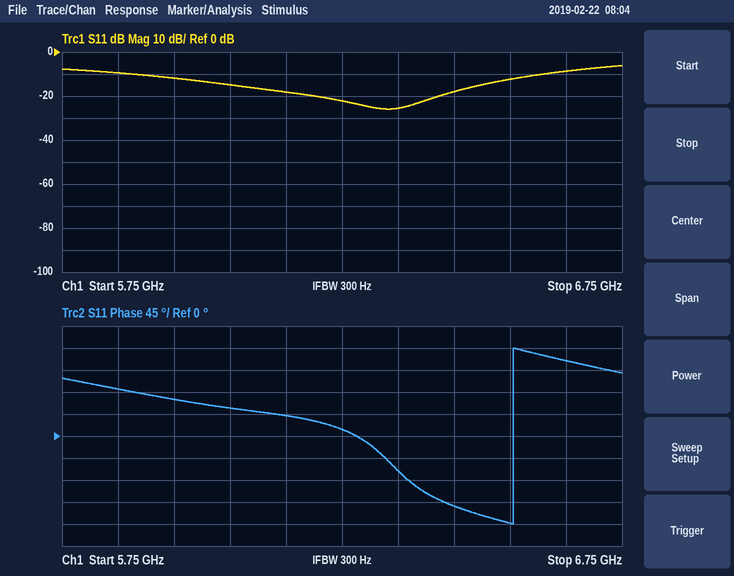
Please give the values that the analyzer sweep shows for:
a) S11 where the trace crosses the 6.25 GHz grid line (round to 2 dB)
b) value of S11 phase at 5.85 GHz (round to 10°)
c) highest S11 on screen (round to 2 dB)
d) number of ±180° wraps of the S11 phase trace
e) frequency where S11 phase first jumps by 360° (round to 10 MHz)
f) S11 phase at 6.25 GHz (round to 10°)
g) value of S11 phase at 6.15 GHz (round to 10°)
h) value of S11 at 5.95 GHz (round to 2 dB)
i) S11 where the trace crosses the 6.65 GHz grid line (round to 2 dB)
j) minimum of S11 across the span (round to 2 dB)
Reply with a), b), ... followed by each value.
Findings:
a) -22 dB
b) 100°
c) -6 dB
d) 1
e) 6.56 GHz
f) 10°
g) 40°
h) -12 dB
i) -8 dB
j) -26 dB
